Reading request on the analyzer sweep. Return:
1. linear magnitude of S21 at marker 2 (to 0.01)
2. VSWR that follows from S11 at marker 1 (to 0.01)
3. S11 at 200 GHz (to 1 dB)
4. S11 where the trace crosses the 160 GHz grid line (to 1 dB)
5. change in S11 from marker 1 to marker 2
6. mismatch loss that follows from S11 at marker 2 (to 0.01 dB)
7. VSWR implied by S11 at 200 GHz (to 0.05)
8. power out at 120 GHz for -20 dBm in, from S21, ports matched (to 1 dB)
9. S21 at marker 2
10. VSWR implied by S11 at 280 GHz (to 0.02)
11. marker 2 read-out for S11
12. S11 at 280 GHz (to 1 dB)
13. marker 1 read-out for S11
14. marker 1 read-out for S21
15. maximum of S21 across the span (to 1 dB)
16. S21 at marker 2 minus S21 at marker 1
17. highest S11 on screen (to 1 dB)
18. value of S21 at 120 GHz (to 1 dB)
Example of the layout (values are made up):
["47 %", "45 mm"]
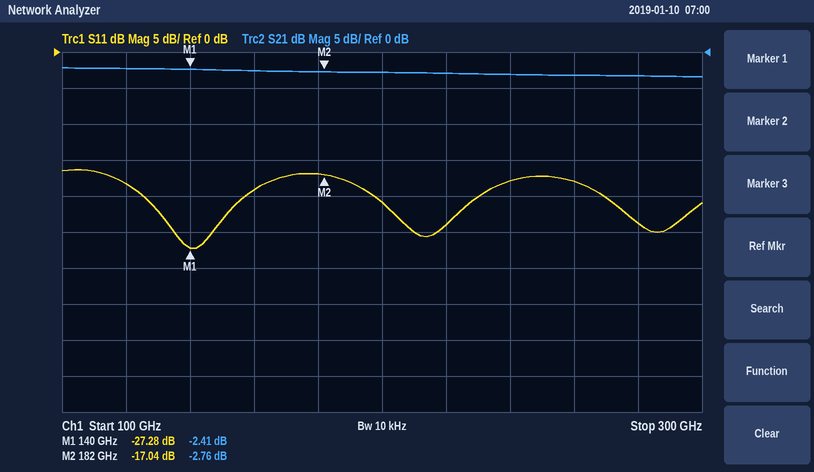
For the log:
["0.73", "1.09", "-21 dB", "-19 dB", "10.24 dB", "0.09 dB", "1.20", "-22 dBm", "-2.76 dB", "1.14", "-17.04 dB", "-24 dB", "-27.28 dB", "-2.41 dB", "-2 dB", "-0.35 dB", "-16 dB", "-2 dB"]
